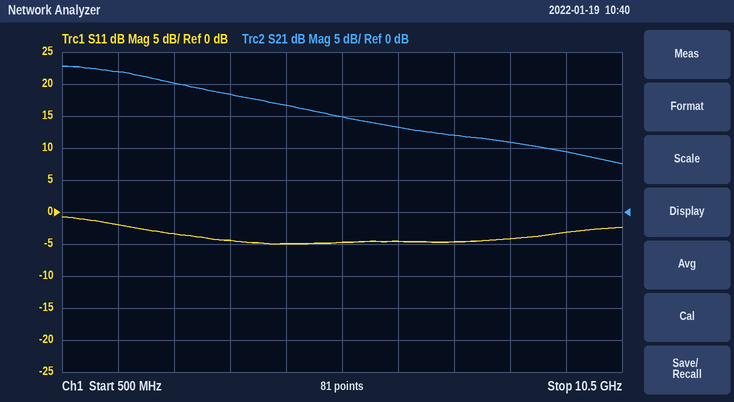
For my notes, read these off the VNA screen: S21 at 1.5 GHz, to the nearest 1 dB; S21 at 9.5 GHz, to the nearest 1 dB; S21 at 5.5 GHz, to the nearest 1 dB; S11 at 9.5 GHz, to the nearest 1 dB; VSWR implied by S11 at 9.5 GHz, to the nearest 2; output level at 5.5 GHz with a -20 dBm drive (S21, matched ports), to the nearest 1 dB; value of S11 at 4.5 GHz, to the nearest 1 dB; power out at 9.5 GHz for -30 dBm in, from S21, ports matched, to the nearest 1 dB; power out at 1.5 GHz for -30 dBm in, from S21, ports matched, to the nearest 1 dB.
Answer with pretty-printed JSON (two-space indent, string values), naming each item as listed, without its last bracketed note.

{
  "S21 at 1.5 GHz, to the nearest 1 dB": "22 dB",
  "S21 at 9.5 GHz, to the nearest 1 dB": "9 dB",
  "S21 at 5.5 GHz, to the nearest 1 dB": "15 dB",
  "S11 at 9.5 GHz, to the nearest 1 dB": "-3 dB",
  "VSWR implied by S11 at 9.5 GHz, to the nearest 2": "6",
  "output level at 5.5 GHz with a -20 dBm drive (S21, matched ports), to the nearest 1 dB": "-5 dBm",
  "value of S11 at 4.5 GHz, to the nearest 1 dB": "-5 dB",
  "power out at 9.5 GHz for -30 dBm in, from S21, ports matched, to the nearest 1 dB": "-21 dBm",
  "power out at 1.5 GHz for -30 dBm in, from S21, ports matched, to the nearest 1 dB": "-8 dBm"
}
